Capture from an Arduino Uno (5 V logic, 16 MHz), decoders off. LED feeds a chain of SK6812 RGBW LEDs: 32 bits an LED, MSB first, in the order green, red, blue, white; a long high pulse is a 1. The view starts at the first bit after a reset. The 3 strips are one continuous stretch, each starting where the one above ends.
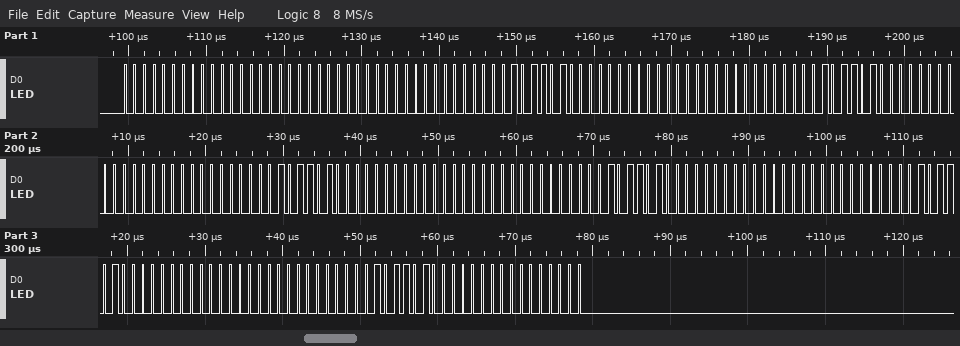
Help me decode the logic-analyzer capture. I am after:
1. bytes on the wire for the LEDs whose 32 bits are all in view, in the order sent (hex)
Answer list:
00 00 00 00 00 B4 00 00 00 B4 00 00 00 B4 00 00 00 2D 00 00 00 2D 00 00 00 2D 00 00
